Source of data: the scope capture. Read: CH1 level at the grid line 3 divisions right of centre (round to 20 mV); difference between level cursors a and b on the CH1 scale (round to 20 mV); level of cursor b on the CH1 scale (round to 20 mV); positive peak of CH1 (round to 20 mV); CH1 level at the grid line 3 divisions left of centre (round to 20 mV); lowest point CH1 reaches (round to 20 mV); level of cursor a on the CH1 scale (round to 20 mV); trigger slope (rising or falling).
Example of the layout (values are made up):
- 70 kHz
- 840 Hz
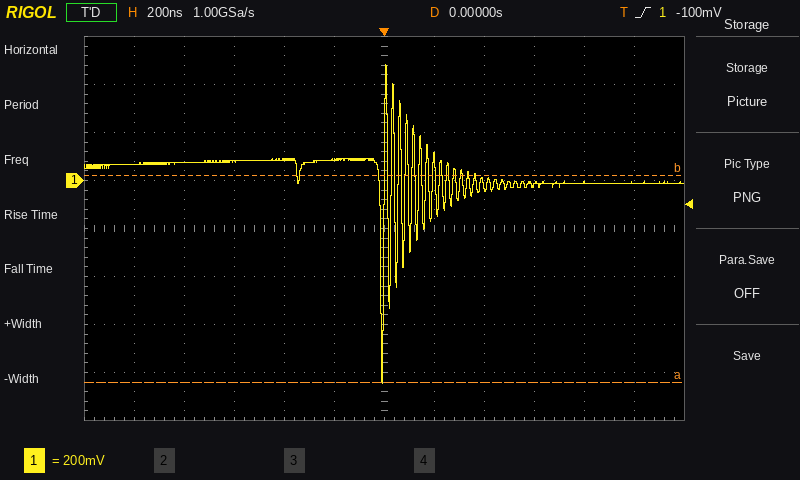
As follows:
- -20 mV
- 860 mV
- 20 mV
- 480 mV
- 80 mV
- -840 mV
- -840 mV
- rising
